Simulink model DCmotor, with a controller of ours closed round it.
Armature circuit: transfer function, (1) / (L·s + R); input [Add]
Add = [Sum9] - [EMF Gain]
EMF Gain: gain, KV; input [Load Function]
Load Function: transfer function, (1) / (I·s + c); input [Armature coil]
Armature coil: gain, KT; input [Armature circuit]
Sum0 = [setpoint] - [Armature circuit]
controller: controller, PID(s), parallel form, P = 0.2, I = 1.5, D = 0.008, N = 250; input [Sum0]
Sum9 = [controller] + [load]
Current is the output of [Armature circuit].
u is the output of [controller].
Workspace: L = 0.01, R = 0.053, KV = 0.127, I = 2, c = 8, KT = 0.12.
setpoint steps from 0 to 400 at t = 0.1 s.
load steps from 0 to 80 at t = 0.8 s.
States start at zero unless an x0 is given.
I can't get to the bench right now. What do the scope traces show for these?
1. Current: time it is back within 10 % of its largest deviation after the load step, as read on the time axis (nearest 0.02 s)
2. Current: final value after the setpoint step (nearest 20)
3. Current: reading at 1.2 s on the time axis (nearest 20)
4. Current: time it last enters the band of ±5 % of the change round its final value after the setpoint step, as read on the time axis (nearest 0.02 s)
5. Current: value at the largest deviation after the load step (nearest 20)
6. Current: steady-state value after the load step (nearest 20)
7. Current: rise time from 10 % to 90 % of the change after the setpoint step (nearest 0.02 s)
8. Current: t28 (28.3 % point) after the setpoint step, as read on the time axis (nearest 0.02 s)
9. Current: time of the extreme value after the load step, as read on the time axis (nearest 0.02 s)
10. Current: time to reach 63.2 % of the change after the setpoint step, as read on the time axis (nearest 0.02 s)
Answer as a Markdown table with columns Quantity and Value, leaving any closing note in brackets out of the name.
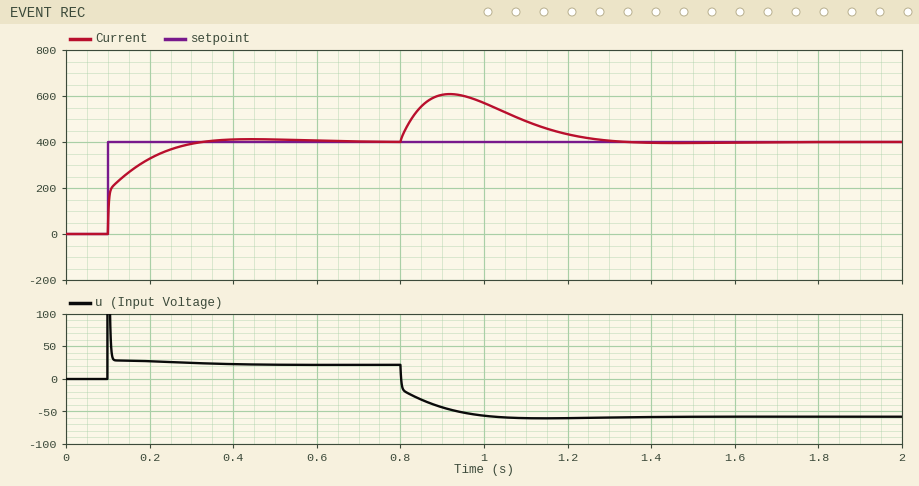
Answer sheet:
| Quantity | Value |
|---|---|
| Current: time it is back within 10 % of its largest deviation after the load step, as read on the time axis | 1.24 s |
| Current: final value after the setpoint step | 400 |
| Current: reading at 1.2 s on the time axis | 440 |
| Current: time it last enters the band of ±5 % of the change round its final value after the setpoint step, as read on the time axis | 0.28 s |
| Current: value at the largest deviation after the load step | 600 |
| Current: steady-state value after the load step | 400 |
| Current: rise time from 10 % to 90 % of the change after the setpoint step | 0.14 s |
| Current: t28 (28.3 % point) after the setpoint step, as read on the time axis | 0.10 s |
| Current: time of the extreme value after the load step, as read on the time axis | 0.92 s |
| Current: time to reach 63.2 % of the change after the setpoint step, as read on the time axis | 0.14 s |
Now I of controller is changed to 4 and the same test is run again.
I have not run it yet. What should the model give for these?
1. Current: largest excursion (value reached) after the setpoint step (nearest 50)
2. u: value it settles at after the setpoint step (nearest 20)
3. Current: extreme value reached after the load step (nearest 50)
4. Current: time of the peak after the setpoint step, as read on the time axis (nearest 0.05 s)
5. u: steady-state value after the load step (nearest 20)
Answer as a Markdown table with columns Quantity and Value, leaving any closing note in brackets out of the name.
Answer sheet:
| Quantity | Value |
|---|---|
| Current: largest excursion (value reached) after the setpoint step | 450 |
| u: value it settles at after the setpoint step | 20 |
| Current: extreme value reached after the load step | 550 |
| Current: time of the peak after the setpoint step, as read on the time axis | 0.30 s |
| u: steady-state value after the load step | -60 |
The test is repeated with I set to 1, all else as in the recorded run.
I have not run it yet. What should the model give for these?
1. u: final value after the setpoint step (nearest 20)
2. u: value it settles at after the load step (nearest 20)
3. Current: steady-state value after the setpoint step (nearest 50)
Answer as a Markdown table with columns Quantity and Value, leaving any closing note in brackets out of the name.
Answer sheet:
| Quantity | Value |
|---|---|
| u: final value after the setpoint step | 20 |
| u: value it settles at after the load step | -60 |
| Current: steady-state value after the setpoint step | 400 |
